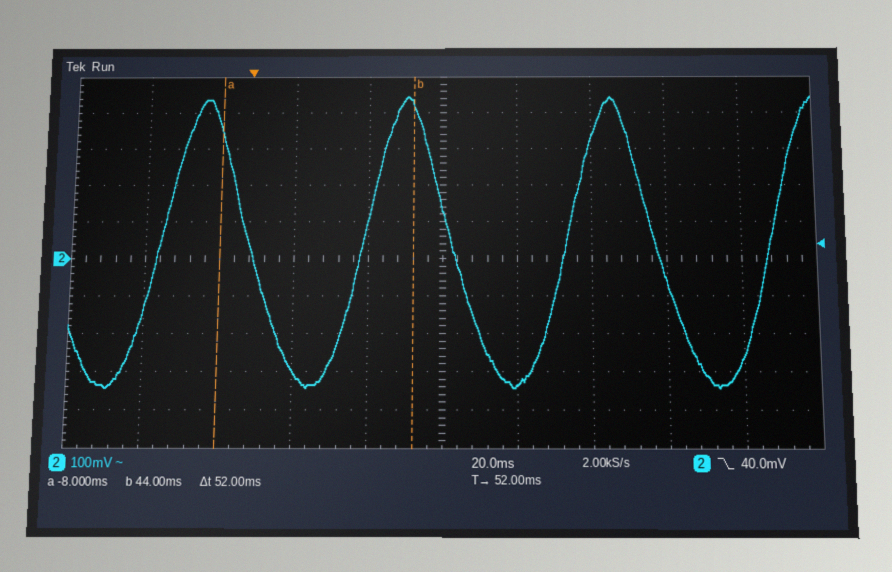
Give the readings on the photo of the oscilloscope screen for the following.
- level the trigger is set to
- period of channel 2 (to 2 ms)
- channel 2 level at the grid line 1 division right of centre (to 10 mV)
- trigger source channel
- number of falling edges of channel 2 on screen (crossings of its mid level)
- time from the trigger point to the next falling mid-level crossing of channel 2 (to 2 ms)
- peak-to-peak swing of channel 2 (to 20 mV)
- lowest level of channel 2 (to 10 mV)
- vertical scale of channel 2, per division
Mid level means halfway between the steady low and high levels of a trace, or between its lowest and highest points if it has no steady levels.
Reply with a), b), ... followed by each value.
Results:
a) 40.0 mV
b) 54 ms
c) -330 mV
d) channel 2
e) 3
f) 54 ms
g) 780 mV
h) -340 mV
i) 100 mV
